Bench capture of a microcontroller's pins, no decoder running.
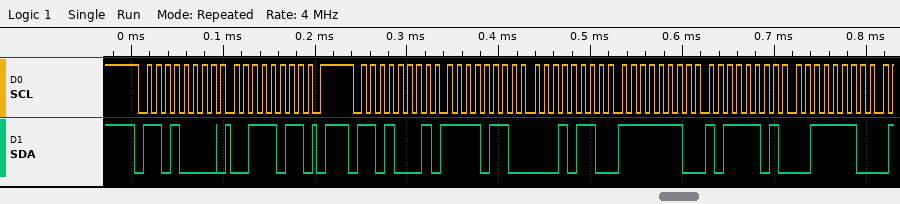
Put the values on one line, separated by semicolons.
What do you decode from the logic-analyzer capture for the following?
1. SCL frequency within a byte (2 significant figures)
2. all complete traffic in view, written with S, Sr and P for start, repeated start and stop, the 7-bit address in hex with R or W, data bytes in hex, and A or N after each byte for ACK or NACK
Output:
100 kHz; S 68W A 3B A P S 68R A F6 A 16 A FE A BD A 3E A
